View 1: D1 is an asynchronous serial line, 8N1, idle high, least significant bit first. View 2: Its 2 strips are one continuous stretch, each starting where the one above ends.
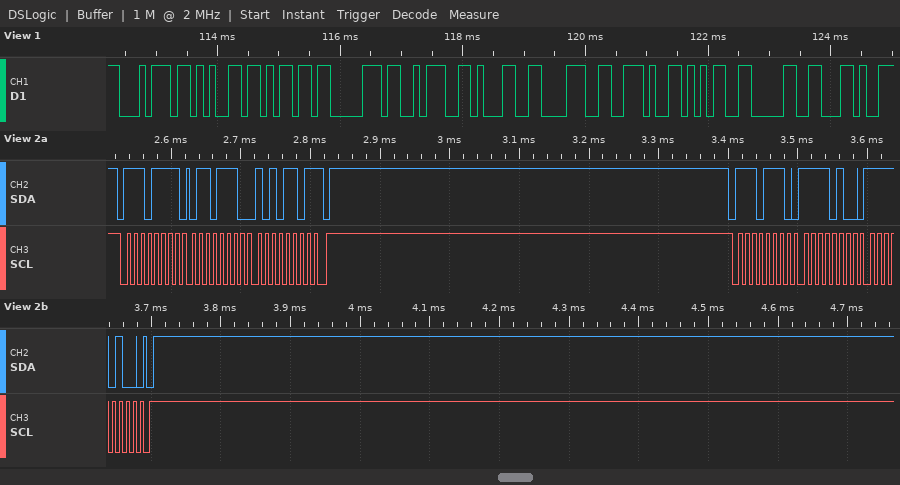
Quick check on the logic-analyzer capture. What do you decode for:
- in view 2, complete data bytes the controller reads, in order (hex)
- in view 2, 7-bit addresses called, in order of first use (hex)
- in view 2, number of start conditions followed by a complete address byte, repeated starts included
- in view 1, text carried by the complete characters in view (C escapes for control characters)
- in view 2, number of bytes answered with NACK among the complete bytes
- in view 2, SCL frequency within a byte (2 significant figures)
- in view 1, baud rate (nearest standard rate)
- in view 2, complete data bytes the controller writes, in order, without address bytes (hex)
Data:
6E AD
0x77
2
"temp:18.50,"
1
100 kHz
9600 baud
F4 F4
